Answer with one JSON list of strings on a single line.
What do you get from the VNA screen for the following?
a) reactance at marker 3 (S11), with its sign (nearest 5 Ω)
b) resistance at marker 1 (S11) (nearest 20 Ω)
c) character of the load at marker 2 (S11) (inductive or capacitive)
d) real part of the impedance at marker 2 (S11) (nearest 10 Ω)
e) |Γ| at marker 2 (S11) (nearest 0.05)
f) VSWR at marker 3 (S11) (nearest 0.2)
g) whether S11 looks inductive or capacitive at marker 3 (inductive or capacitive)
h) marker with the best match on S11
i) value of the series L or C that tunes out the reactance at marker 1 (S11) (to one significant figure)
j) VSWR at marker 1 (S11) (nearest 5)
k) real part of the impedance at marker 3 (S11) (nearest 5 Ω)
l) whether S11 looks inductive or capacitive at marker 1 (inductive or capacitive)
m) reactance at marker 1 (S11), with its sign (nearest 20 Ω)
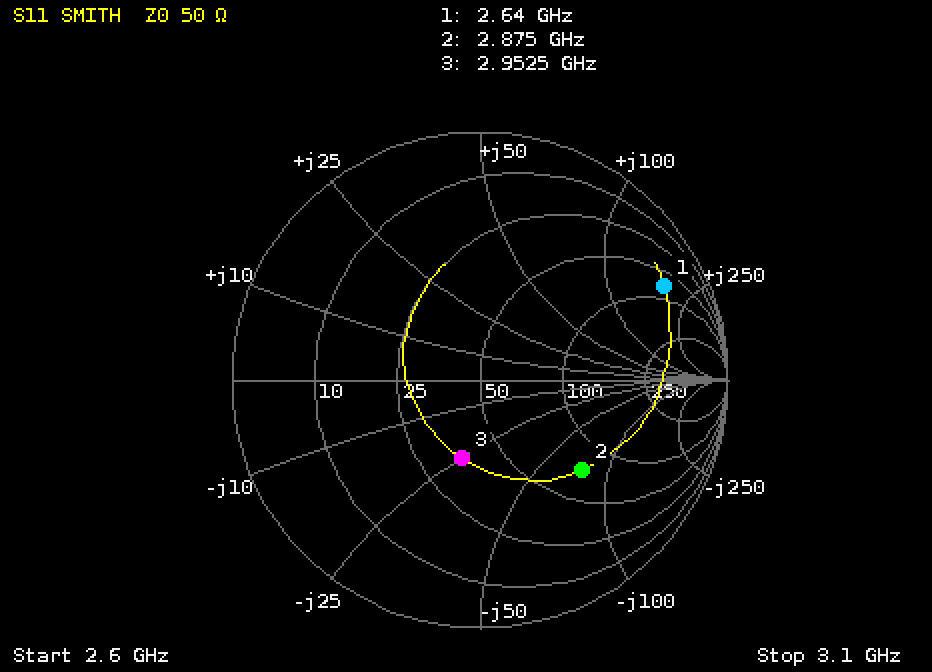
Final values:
["-25 Ω", "80 Ω", "capacitive", "70 Ω", "0.55", "2.0", "capacitive", "marker 3", "300 fF", "10", "35 Ω", "inductive", "+180 Ω"]
